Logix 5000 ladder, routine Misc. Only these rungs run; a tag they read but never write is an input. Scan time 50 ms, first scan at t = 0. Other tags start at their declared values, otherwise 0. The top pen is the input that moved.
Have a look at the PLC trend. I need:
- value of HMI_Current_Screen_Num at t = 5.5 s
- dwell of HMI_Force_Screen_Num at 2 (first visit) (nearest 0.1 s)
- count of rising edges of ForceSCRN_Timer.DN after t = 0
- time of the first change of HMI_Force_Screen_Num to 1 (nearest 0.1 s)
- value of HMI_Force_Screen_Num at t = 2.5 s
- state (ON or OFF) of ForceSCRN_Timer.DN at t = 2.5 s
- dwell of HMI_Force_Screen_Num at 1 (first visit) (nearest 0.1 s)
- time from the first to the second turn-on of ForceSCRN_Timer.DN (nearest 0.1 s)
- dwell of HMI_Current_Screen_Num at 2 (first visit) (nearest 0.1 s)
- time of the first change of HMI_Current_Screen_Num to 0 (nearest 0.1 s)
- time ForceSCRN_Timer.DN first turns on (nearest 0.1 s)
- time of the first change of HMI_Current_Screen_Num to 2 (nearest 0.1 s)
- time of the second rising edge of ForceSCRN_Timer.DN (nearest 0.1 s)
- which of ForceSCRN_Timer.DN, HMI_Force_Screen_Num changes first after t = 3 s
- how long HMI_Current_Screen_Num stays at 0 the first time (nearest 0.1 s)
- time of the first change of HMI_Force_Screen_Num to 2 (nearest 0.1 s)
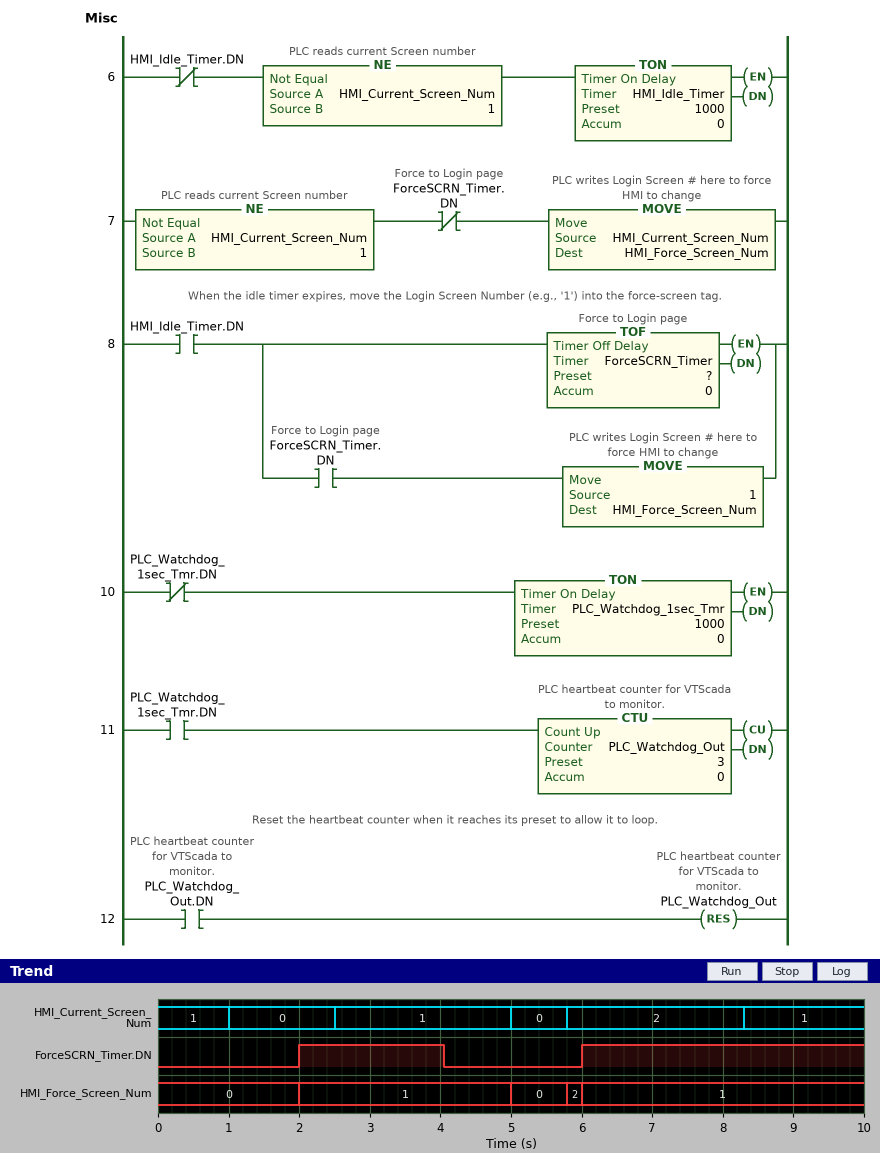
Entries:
0
0.2 s
2
2.0 s
1
ON
3.0 s
4.0 s
2.5 s
1.0 s
2.0 s
5.8 s
6.0 s
ForceSCRN_Timer.DN
1.5 s
5.8 s
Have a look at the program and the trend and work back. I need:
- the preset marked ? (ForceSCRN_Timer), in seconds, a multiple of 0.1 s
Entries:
2.0 s
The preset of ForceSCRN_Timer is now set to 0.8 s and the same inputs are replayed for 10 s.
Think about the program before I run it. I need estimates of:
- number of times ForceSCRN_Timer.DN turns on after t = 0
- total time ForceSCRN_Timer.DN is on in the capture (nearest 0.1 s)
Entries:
4
3.4 s
